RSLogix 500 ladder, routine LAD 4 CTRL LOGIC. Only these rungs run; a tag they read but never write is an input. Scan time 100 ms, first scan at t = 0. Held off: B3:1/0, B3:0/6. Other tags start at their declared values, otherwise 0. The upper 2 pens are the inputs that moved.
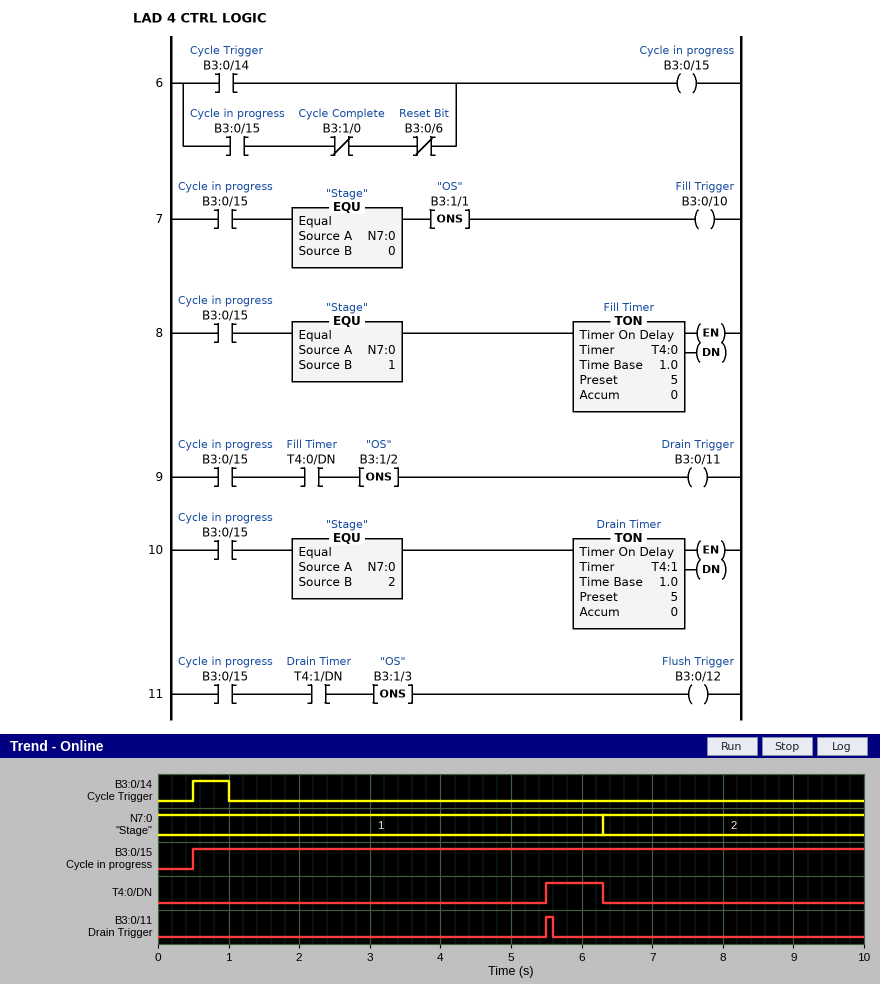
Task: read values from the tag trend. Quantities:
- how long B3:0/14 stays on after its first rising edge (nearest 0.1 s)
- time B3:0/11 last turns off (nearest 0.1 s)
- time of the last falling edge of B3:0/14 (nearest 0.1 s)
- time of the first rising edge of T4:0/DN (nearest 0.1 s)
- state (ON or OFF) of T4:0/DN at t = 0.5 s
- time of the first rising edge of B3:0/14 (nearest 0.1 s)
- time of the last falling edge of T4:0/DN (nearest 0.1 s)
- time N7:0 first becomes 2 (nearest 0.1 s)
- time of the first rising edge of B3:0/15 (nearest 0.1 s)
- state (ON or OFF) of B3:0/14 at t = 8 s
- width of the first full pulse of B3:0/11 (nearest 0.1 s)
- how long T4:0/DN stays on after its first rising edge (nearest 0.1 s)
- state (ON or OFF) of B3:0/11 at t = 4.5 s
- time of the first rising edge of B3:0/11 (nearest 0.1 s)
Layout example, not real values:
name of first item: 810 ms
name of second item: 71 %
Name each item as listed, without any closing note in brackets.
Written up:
how long B3:0/14 stays on after its first rising edge: 0.5 s
time B3:0/11 last turns off: 5.6 s
time of the last falling edge of B3:0/14: 1.0 s
time of the first rising edge of T4:0/DN: 5.5 s
state (ON or OFF) of T4:0/DN at t = 0.5 s: OFF
time of the first rising edge of B3:0/14: 0.5 s
time of the last falling edge of T4:0/DN: 6.3 s
time N7:0 first becomes 2: 6.3 s
time of the first rising edge of B3:0/15: 0.5 s
state (ON or OFF) of B3:0/14 at t = 8 s: OFF
width of the first full pulse of B3:0/11: 0.1 s
how long T4:0/DN stays on after its first rising edge: 0.8 s
state (ON or OFF) of B3:0/11 at t = 4.5 s: OFF
time of the first rising edge of B3:0/11: 5.5 s
